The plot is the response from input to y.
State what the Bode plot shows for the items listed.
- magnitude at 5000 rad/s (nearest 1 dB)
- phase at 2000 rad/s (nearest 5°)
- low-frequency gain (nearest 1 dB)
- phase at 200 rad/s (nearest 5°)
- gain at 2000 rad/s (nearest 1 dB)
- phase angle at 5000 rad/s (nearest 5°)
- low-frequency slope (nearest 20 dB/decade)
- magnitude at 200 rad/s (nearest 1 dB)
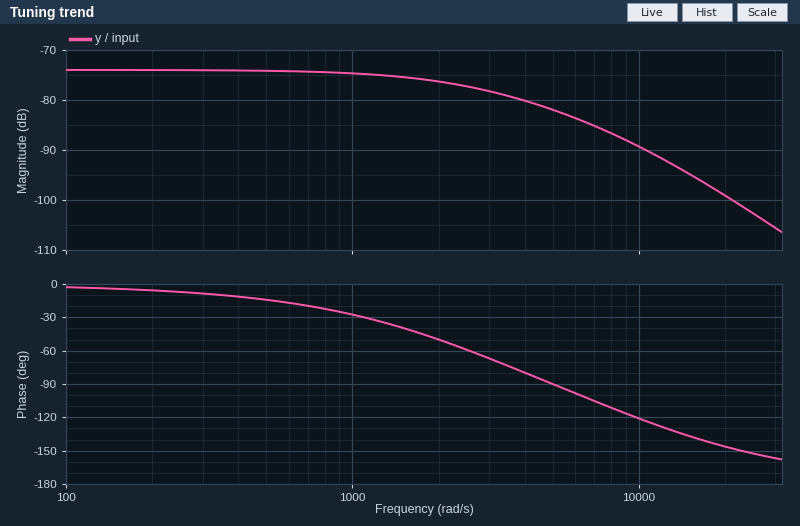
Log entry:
-82 dB
-50°
-74 dB
-5°
-76 dB
-90°
0 dB/decade
-74 dB
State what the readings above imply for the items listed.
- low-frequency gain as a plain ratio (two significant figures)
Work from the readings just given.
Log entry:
0.00020
